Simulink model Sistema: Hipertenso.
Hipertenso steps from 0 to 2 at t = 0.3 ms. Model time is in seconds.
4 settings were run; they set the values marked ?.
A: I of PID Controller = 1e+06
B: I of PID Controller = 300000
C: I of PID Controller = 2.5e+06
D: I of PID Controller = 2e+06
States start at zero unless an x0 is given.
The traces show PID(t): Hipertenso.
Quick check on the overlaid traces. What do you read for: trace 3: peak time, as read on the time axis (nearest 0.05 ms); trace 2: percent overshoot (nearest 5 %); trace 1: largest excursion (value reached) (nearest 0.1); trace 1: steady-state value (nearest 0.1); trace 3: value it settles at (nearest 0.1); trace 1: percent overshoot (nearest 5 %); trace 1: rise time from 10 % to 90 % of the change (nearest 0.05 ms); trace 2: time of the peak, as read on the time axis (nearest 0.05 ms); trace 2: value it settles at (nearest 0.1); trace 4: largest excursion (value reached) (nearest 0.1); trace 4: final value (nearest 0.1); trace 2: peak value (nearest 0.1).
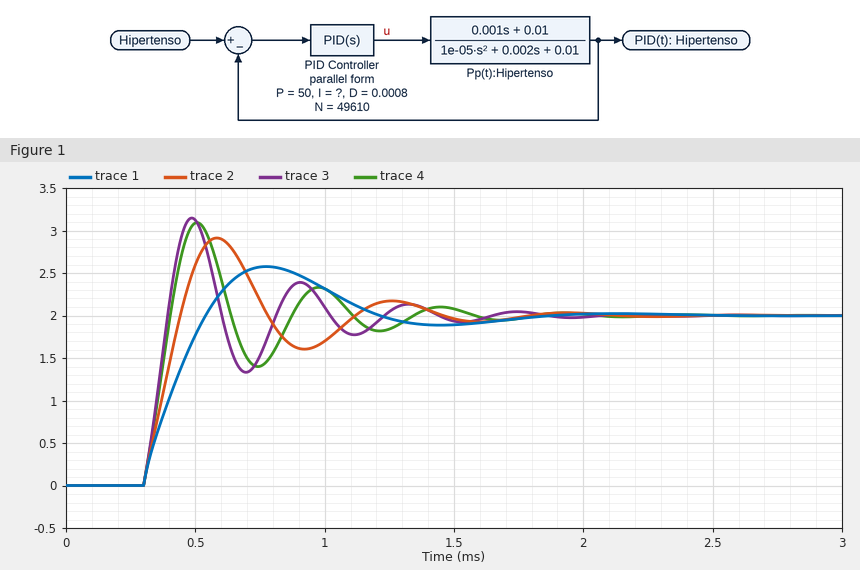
0.50 ms
45 %
2.6
2.0
2.0
30 %
0.20 ms
0.60 ms
2.0
3.1
2.0
2.9
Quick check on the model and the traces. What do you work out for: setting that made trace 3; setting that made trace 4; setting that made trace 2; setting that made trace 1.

C
D
A
B
